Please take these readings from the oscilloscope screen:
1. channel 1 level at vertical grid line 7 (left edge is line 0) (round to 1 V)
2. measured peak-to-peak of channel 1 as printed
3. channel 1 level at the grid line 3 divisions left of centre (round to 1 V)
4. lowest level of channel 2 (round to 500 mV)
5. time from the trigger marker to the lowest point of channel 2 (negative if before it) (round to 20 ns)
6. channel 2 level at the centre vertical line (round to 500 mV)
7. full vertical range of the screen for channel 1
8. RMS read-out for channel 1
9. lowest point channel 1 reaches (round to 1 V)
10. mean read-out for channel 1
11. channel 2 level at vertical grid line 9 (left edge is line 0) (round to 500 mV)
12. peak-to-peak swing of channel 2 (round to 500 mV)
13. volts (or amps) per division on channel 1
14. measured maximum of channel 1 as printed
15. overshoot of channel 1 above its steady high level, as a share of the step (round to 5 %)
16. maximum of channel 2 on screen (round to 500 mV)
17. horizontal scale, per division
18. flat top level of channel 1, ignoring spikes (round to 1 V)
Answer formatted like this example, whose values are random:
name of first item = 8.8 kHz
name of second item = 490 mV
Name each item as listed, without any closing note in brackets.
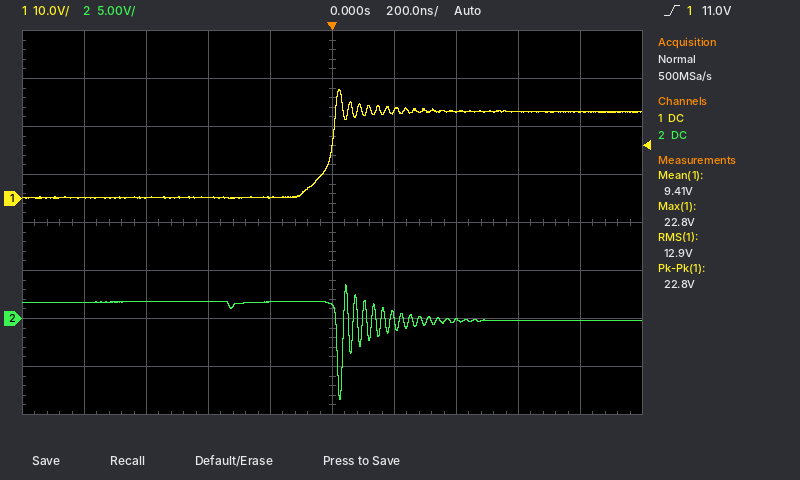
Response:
channel 1 level at vertical grid line 7 (left edge is line 0) = 18 V
measured peak-to-peak of channel 1 as printed = 22.8 V
channel 1 level at the grid line 3 divisions left of centre = 0 V
lowest level of channel 2 = -8.5 V
time from the trigger marker to the lowest point of channel 2 (negative if before it) = +20 ns
channel 2 level at the centre vertical line = 1.0 V
full vertical range of the screen for channel 1 = 80 V
RMS read-out for channel 1 = 12.9 V
lowest point channel 1 reaches = 0 V
mean read-out for channel 1 = 9.41 V
channel 2 level at vertical grid line 9 (left edge is line 0) = 0.0 V
peak-to-peak swing of channel 2 = 12.0 V
volts (or amps) per division on channel 1 = 10 V
measured maximum of channel 1 as printed = 22.8 V
overshoot of channel 1 above its steady high level, as a share of the step = 25 %
maximum of channel 2 on screen = 3.5 V
horizontal scale, per division = 200 ns
flat top level of channel 1, ignoring spikes = 18 V
